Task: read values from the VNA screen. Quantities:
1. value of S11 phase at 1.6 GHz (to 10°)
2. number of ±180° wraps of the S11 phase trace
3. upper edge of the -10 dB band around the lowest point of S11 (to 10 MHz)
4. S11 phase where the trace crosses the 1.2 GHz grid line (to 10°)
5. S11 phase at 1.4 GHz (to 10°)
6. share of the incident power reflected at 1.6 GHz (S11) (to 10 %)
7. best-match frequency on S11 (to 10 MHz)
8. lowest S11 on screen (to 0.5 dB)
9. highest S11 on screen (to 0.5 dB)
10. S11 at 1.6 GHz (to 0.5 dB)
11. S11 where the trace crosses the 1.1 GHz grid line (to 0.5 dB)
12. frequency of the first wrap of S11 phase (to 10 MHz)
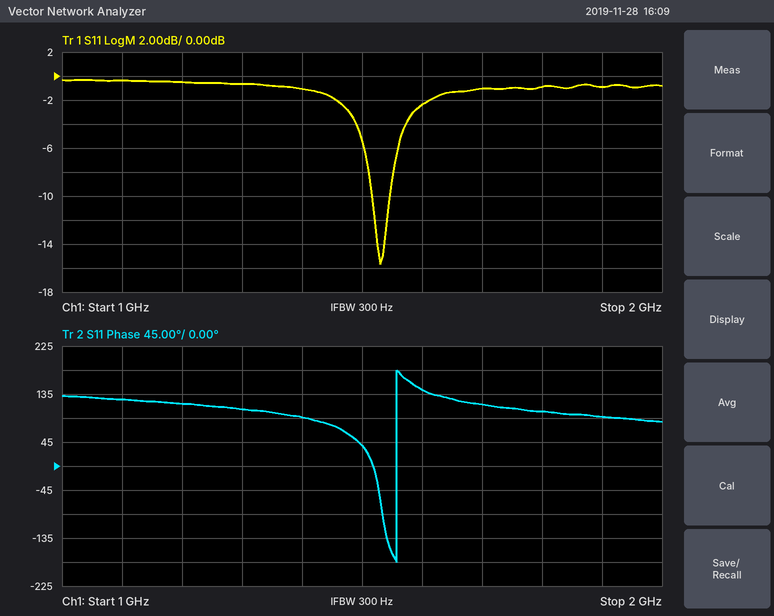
140°
1
1.55 GHz
120°
90°
60 %
1.53 GHz
-15.5 dB
-0.5 dB
-2.5 dB
-0.5 dB
1.56 GHz
